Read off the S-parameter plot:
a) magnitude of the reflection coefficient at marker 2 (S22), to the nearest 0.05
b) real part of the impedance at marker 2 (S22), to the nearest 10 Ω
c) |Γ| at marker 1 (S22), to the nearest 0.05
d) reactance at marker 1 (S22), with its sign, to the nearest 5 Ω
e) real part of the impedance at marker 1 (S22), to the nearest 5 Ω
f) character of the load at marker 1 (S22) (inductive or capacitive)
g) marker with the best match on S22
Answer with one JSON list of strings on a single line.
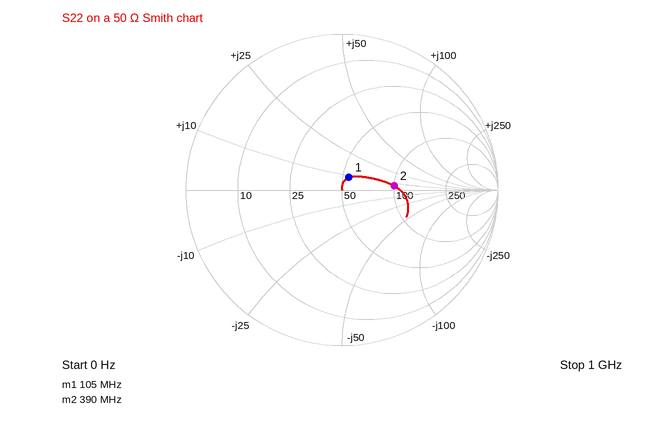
["0.35", "100 Ω", "0.10", "+10 Ω", "55 Ω", "inductive", "marker 1"]
